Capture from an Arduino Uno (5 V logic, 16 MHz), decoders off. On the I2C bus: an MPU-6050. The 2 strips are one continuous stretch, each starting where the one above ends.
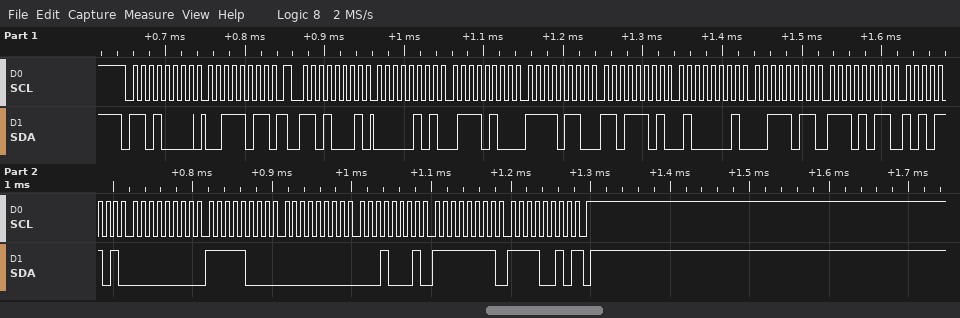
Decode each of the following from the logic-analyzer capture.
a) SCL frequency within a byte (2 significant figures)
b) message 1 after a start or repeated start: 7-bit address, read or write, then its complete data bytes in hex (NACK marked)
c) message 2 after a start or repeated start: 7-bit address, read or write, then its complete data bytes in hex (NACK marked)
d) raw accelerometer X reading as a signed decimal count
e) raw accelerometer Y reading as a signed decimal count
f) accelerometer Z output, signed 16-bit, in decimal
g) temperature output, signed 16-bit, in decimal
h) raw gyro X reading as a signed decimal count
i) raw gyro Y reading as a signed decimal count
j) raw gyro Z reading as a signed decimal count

100 kHz
0x68 write: 3B
0x68 read: 05 74 F6 DD 41 3B EB AD 00 F8 00 11 FF F2 NACK
1396
-2339
16699
-5203
248
17
-14
